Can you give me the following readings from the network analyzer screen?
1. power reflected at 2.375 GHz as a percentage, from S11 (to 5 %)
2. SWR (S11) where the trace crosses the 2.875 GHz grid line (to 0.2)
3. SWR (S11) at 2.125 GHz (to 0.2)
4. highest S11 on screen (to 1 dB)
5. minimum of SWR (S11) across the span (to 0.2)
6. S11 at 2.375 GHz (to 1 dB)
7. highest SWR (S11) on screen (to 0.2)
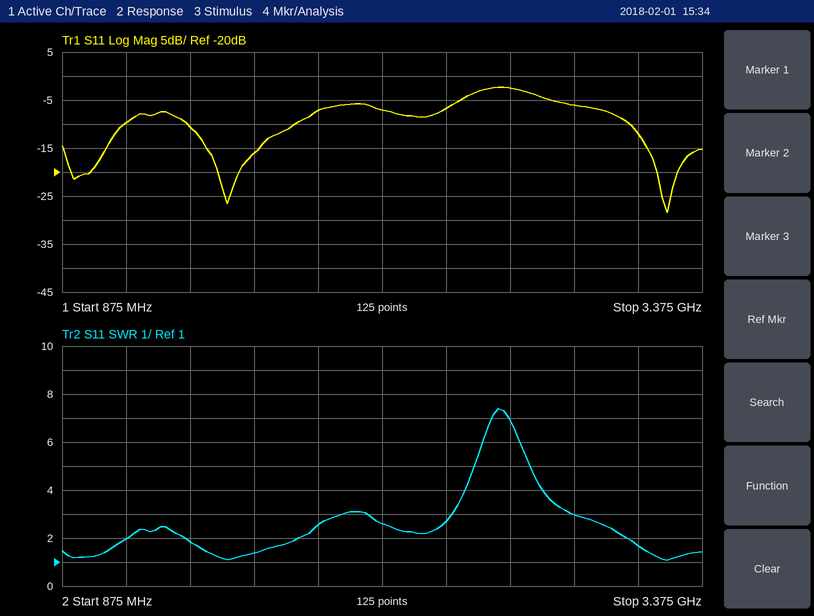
20 %
3.0
2.6
-2 dB
1.0
-7 dB
7.4
